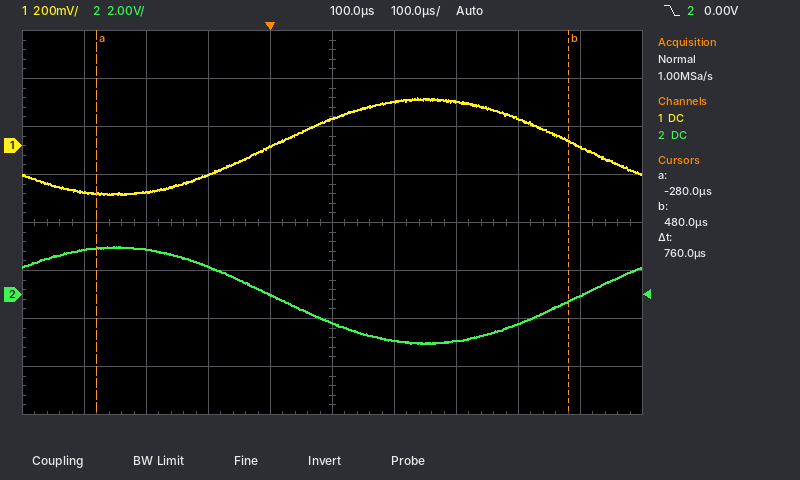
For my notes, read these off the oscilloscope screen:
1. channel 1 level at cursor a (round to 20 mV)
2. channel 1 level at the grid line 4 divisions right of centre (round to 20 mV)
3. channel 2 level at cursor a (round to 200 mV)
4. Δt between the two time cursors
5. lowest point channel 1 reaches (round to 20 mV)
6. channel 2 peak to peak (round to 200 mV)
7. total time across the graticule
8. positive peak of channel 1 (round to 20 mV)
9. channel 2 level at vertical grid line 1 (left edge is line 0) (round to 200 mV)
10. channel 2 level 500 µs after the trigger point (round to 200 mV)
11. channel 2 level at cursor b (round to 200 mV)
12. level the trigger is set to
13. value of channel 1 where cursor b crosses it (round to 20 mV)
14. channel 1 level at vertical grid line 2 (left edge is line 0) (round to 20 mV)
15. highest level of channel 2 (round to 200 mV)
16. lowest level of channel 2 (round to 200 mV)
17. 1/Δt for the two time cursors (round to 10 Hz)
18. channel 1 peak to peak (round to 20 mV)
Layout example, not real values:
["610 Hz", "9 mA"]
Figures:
["-200 mV", "0 mV", "2.0 V", "760 µs", "-200 mV", "4.0 V", "1 ms", "200 mV", "1.8 V", "0.0 V", "-200 mV", "0.00 V", "20 mV", "-200 mV", "2.0 V", "-2.0 V", "1.32 kHz", "400 mV"]
